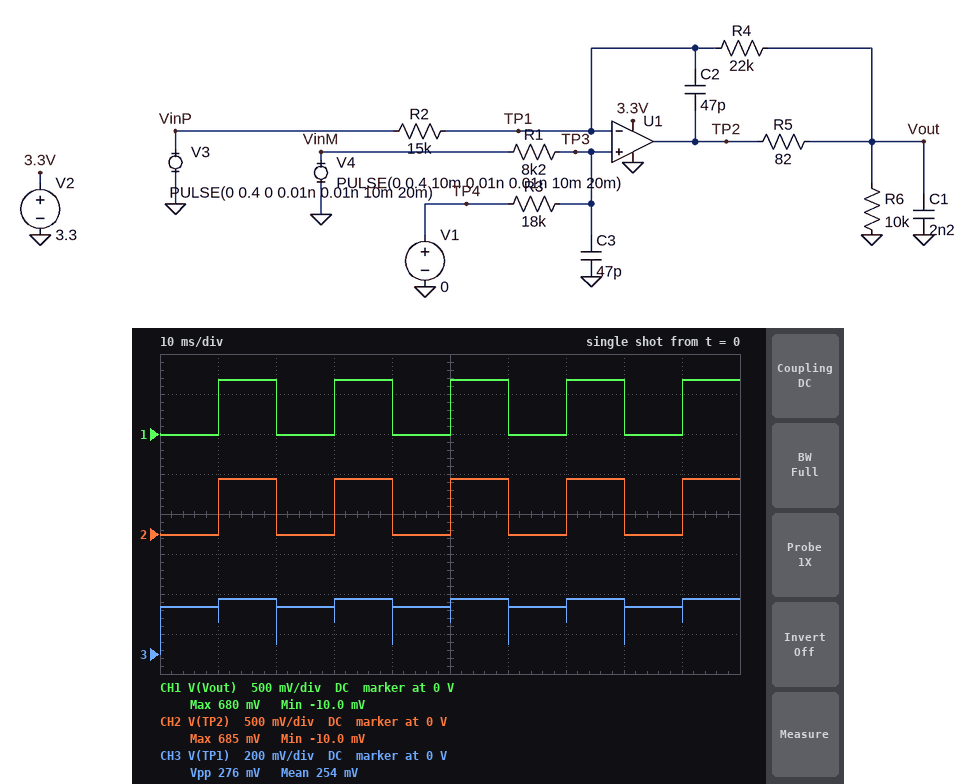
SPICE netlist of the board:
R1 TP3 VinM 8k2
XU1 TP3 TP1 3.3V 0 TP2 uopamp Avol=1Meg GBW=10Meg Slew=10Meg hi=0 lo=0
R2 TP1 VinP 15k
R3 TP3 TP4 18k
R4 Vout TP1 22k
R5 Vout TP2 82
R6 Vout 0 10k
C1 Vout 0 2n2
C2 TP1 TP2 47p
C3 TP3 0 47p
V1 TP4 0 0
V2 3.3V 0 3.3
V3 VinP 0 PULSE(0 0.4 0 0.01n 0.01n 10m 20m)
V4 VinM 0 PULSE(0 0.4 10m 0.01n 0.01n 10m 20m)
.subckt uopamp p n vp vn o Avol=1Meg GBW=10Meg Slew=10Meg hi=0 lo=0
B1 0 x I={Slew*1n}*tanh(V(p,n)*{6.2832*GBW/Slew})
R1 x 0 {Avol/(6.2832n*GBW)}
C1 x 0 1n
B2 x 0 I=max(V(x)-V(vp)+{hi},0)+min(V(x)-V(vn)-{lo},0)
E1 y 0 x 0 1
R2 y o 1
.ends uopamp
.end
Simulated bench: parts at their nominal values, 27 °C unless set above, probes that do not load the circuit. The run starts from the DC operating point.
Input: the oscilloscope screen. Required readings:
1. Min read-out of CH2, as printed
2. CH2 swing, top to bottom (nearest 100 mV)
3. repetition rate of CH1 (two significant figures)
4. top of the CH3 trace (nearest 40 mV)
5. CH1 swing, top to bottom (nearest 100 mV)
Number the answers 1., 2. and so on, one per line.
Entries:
1. -10.0 mV
2. 700 mV
3. 50 Hz
4. 280 mV
5. 700 mV
